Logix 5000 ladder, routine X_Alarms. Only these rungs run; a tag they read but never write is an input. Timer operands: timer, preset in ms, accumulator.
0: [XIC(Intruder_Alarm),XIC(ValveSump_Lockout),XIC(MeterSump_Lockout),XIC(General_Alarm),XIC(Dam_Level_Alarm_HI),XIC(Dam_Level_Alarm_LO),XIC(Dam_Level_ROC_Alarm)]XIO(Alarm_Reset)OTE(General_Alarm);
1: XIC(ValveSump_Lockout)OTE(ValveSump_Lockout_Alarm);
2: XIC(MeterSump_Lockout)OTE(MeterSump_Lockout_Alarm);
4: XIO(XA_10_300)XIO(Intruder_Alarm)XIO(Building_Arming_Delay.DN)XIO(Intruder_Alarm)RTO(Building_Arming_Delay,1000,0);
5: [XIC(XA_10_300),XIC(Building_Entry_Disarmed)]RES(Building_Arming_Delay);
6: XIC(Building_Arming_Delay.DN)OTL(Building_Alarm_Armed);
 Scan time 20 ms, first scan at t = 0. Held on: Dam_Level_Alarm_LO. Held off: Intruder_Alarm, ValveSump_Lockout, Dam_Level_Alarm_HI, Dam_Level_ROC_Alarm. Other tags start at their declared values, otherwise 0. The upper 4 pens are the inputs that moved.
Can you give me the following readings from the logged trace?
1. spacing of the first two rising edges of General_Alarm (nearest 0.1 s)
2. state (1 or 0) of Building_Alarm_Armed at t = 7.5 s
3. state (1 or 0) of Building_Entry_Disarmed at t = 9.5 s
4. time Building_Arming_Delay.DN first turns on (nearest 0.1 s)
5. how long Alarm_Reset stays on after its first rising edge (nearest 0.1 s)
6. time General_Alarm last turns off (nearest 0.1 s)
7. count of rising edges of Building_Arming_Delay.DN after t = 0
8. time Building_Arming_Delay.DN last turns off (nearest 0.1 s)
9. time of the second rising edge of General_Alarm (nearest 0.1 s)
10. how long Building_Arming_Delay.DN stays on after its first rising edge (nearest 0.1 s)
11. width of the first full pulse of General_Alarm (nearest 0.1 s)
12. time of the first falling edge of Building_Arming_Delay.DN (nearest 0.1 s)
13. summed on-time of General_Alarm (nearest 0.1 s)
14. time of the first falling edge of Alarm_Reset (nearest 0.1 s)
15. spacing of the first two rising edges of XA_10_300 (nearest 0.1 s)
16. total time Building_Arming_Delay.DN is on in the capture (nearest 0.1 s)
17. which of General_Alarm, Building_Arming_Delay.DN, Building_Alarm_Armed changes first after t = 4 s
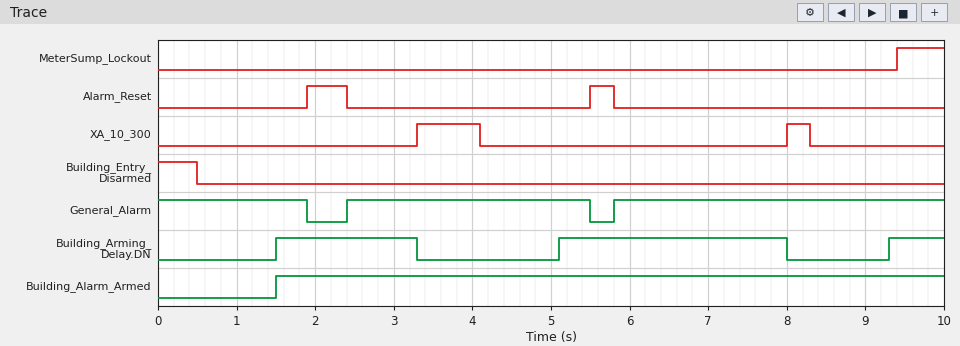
3.4 s
1
0
1.5 s
0.5 s
5.5 s
3
8.0 s
5.8 s
1.8 s
3.1 s
3.3 s
9.2 s
2.4 s
4.7 s
5.4 s
Building_Arming_Delay.DN
